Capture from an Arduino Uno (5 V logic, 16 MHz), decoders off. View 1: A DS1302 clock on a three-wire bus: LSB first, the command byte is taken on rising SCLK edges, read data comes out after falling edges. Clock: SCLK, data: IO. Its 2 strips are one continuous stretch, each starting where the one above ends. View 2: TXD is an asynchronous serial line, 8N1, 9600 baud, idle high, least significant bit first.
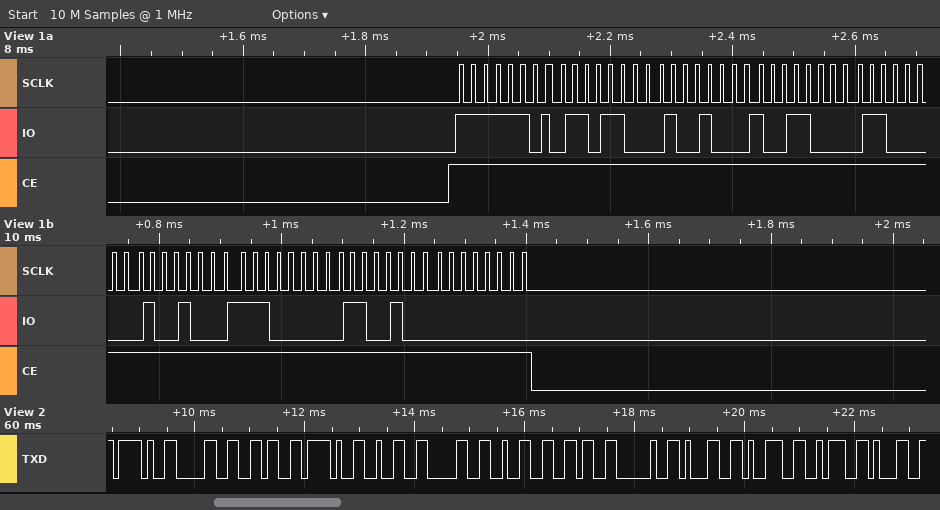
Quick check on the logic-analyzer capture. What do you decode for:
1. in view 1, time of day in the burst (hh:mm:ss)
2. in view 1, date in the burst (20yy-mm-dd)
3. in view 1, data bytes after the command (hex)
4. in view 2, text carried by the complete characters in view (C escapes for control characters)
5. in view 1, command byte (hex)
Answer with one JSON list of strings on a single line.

["19:12:36", "2026-12-06", "36 12 19 06 12 07 26 00", "\"/06/2026 19:1\"", "0xBF"]
